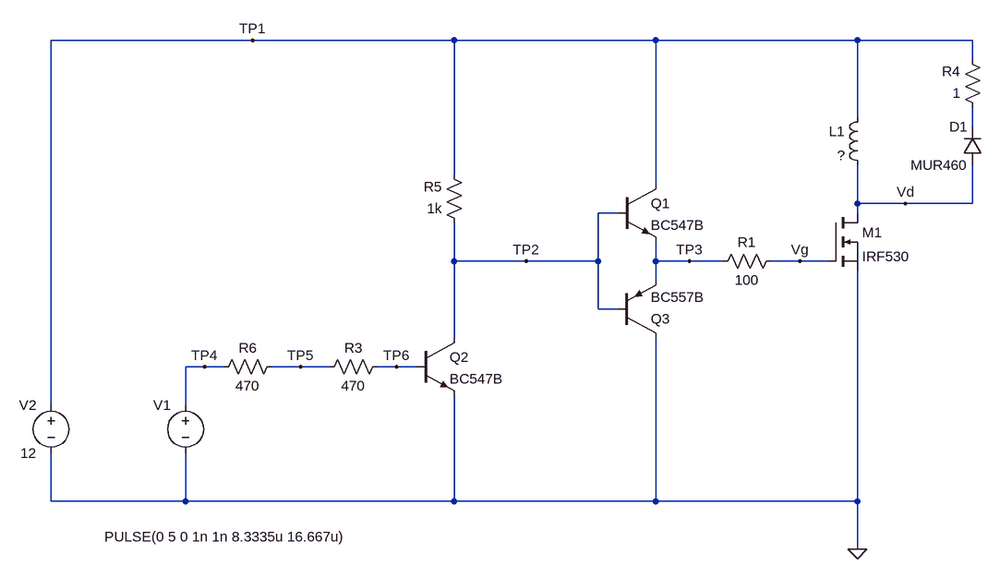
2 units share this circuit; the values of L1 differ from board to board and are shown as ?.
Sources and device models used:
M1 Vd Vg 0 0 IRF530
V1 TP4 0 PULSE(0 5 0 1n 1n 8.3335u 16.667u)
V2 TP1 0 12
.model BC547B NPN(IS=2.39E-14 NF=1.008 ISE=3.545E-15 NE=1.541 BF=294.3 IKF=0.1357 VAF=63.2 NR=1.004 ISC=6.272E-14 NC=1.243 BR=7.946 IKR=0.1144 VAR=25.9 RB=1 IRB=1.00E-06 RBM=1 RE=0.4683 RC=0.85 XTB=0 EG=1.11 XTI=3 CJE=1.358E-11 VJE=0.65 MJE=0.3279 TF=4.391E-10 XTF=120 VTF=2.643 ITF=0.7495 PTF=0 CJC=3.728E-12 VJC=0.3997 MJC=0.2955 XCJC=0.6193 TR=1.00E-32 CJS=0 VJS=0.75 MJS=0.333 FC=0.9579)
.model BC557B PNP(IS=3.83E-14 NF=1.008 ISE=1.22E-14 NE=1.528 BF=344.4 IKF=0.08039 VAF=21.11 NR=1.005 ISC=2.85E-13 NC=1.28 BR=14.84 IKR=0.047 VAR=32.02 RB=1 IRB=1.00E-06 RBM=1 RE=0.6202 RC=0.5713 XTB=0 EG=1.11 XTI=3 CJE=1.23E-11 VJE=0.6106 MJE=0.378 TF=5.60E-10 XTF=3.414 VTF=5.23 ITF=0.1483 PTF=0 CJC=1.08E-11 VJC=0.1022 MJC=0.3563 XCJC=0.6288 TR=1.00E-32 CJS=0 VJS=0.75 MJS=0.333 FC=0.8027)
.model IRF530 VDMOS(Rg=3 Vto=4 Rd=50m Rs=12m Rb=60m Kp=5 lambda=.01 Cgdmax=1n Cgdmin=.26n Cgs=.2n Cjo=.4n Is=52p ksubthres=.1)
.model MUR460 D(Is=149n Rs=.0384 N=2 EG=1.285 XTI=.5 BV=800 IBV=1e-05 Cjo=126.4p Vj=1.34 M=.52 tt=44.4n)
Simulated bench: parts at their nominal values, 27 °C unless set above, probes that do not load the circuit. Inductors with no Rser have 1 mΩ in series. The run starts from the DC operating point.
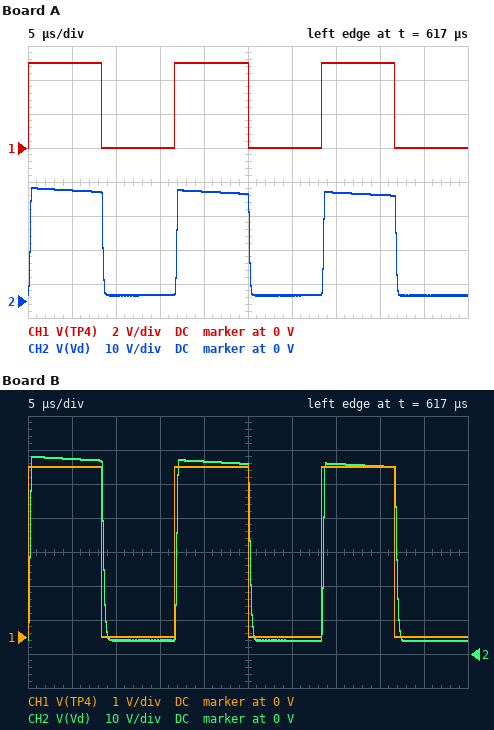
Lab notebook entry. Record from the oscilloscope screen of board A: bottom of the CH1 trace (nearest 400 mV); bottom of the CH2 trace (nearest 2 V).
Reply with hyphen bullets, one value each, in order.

- 0 V
- 2 V
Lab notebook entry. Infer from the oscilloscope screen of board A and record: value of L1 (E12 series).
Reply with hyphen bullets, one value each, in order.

- 150 µH
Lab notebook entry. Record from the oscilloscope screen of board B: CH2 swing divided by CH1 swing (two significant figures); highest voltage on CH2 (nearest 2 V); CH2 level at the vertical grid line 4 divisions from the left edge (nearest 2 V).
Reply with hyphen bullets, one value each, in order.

- 11
- 58 V
- 56 V
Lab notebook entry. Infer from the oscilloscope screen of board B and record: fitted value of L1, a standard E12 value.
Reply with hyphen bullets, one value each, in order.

- 330 µH
